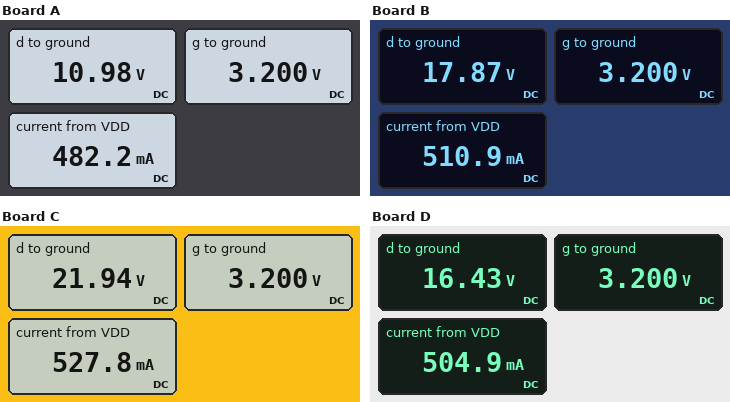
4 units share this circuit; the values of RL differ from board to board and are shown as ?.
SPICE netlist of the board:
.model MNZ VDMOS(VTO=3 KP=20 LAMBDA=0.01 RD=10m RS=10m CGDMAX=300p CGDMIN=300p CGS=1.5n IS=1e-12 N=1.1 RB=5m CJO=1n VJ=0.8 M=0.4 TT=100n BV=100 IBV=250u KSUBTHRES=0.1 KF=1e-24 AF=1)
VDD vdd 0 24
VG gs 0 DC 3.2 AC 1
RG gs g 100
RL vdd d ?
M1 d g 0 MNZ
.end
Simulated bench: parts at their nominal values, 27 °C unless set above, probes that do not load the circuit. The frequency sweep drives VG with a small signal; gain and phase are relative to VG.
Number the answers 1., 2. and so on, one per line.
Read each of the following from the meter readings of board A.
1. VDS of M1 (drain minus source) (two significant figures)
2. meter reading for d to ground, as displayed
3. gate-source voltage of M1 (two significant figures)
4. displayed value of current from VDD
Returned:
1. 11 V
2. 10.98 V
3. 3.2 V
4. 482.2 mA
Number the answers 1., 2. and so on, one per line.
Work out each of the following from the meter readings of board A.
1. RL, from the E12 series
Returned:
1. 27 Ω
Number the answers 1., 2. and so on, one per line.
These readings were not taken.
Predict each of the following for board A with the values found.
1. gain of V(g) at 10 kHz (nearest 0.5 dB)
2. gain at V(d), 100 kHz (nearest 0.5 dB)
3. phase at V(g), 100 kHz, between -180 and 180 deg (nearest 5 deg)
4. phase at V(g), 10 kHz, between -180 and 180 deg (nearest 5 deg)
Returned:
1. 0 dB
2. 33.0 dB
3. -60 deg
4. -10 deg
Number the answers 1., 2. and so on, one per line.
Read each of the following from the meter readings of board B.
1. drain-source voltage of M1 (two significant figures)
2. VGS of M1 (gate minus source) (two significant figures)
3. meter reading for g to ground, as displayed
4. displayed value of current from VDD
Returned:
1. 18 V
2. 3.2 V
3. 3.200 V
4. 510.9 mA
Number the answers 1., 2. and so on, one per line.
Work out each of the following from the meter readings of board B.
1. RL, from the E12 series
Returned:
1. 12 Ω
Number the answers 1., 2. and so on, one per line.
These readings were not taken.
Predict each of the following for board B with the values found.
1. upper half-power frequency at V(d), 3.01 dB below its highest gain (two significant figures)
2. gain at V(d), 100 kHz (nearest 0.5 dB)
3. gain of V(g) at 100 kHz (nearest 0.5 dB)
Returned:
1. 100 kHz
2. 30.5 dB
3. -3.0 dB
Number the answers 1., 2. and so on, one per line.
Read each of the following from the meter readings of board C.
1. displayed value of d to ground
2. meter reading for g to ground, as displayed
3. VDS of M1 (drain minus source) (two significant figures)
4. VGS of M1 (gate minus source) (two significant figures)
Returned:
1. 21.94 V
2. 3.200 V
3. 22 V
4. 3.2 V
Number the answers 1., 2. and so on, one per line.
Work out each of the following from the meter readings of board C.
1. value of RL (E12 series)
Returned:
1. 3.9 Ω
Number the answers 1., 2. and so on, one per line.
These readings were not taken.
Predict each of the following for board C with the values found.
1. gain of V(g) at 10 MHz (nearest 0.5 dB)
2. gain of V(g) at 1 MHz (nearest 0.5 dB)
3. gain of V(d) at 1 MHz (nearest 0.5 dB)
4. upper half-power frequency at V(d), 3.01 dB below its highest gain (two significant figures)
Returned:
1. -32.5 dB
2. -12.5 dB
3. 11.5 dB
4. 240 kHz
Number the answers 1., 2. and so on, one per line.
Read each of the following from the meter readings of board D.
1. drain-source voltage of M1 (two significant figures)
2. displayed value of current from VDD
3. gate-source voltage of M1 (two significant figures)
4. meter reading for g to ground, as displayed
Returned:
1. 16 V
2. 504.9 mA
3. 3.2 V
4. 3.200 V
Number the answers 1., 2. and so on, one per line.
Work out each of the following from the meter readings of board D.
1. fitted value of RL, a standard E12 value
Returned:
1. 15 Ω
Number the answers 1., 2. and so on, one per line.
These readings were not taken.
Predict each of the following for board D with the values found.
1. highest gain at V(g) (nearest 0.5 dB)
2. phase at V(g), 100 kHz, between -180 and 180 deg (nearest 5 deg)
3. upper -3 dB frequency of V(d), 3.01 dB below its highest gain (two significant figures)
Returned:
1. 0 dB
2. -50 deg
3. 83 kHz
